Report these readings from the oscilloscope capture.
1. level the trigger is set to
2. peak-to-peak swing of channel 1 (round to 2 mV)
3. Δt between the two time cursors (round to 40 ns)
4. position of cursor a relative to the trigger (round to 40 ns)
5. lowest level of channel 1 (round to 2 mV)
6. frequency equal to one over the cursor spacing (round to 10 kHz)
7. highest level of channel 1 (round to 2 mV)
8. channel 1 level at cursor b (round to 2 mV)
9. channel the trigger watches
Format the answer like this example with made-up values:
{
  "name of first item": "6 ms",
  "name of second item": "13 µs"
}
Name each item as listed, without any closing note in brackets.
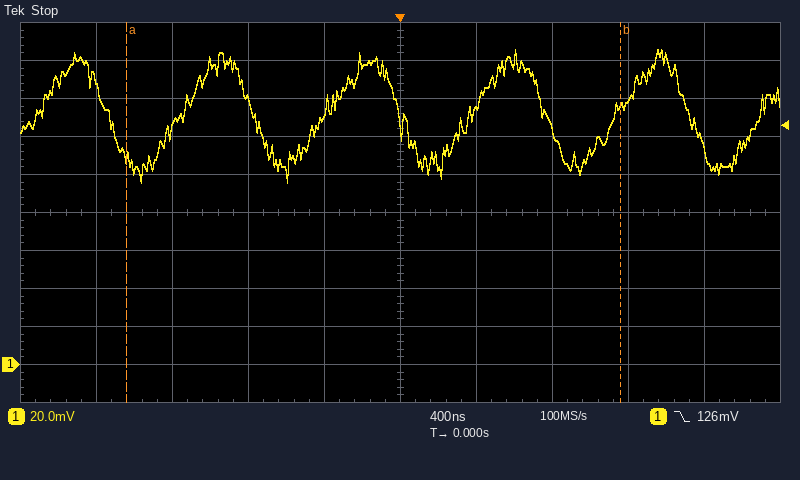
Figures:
{
  "level the trigger is set to": "126 mV",
  "peak-to-peak swing of channel 1": "70 mV",
  "Δt between the two time cursors": "2.60 µs",
  "position of cursor a relative to the trigger": "-1.44 µs",
  "lowest level of channel 1": "96 mV",
  "frequency equal to one over the cursor spacing": "380 kHz",
  "highest level of channel 1": "166 mV",
  "channel 1 level at cursor b": "136 mV",
  "channel the trigger watches": "channel 1"
}
